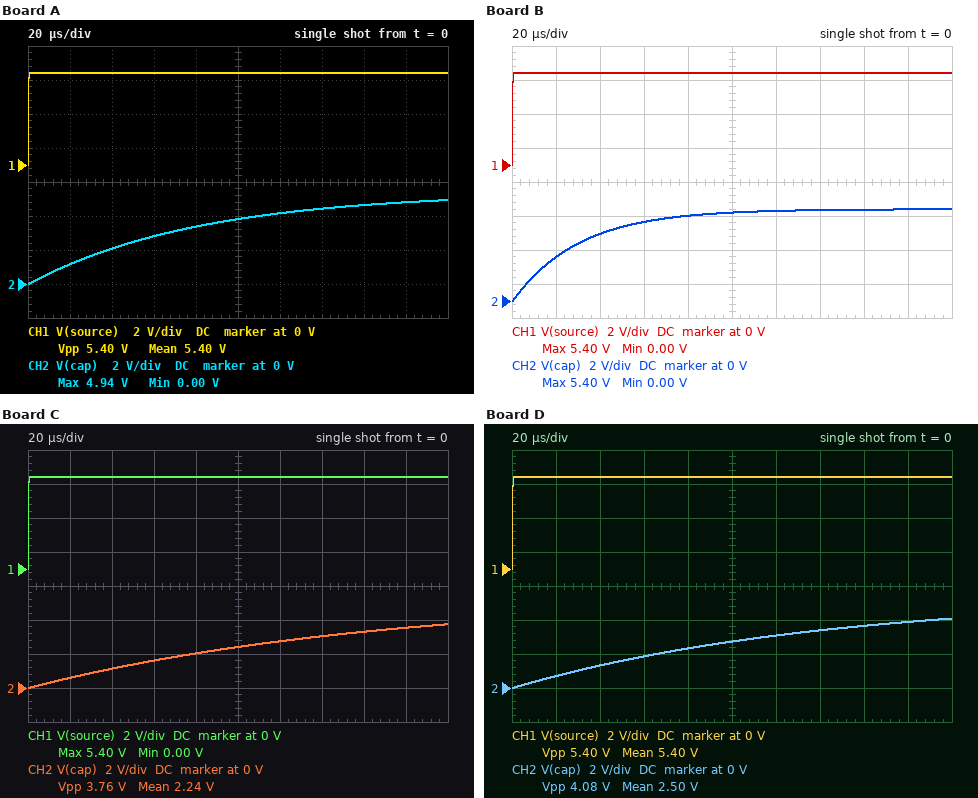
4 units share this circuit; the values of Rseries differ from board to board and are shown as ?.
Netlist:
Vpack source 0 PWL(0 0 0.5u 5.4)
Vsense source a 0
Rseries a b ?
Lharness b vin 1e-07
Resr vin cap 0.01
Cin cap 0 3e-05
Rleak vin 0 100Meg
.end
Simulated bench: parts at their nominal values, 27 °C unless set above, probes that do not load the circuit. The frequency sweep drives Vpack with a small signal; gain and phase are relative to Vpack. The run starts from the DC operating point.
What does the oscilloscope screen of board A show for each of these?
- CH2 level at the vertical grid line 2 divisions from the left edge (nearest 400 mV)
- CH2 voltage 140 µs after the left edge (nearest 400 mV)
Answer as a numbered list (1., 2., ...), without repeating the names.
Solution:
1. 2.0 V
2. 4.4 V
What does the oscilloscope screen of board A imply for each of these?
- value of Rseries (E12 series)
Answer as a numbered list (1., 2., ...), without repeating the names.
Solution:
1. 2.7 Ω
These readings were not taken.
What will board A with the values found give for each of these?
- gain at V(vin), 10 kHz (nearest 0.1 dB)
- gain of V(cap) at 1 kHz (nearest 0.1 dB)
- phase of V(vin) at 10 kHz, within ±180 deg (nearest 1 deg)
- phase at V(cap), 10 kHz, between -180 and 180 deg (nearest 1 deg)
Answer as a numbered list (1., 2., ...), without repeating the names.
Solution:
1. -14.3 dB
2. -1.0 dB
3. -78 deg
4. -79 deg
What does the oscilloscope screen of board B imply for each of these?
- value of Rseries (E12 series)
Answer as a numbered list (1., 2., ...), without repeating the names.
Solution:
1. 1 Ω
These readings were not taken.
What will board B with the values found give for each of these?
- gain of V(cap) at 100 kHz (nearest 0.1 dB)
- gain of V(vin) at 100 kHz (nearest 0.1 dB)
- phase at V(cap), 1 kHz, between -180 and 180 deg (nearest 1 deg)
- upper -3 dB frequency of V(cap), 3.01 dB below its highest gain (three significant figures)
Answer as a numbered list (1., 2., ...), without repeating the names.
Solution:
1. -25.6 dB
2. -25.4 dB
3. -11 deg
4. 5.27 kHz
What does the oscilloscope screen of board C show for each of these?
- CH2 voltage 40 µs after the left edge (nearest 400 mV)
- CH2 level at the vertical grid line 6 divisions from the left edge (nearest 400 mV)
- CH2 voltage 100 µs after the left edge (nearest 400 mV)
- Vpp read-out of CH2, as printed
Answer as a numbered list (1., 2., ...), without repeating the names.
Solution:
1. 1.2 V
2. 2.8 V
3. 2.4 V
4. 3.76 V
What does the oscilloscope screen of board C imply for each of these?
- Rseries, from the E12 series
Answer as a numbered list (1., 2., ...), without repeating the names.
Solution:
1. 5.6 Ω
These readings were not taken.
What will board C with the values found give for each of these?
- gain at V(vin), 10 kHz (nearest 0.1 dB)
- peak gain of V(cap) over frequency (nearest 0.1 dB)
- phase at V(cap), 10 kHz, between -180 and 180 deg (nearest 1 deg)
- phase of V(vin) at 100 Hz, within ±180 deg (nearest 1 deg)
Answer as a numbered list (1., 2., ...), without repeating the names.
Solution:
1. -20.5 dB
2. 0 dB
3. -85 deg
4. -6 deg
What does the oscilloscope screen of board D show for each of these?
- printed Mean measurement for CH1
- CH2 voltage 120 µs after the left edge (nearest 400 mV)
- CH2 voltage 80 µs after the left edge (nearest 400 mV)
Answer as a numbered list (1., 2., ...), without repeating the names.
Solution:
1. 5.40 V
2. 3.2 V
3. 2.4 V
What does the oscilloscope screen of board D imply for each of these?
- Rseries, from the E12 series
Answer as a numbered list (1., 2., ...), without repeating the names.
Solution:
1. 4.7 Ω
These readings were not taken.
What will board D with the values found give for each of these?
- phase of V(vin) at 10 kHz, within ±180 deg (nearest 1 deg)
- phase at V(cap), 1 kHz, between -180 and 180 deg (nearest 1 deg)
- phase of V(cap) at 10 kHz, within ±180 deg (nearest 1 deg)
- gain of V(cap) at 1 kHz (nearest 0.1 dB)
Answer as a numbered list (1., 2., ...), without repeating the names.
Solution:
1. -83 deg
2. -42 deg
3. -84 deg
4. -2.5 dB
